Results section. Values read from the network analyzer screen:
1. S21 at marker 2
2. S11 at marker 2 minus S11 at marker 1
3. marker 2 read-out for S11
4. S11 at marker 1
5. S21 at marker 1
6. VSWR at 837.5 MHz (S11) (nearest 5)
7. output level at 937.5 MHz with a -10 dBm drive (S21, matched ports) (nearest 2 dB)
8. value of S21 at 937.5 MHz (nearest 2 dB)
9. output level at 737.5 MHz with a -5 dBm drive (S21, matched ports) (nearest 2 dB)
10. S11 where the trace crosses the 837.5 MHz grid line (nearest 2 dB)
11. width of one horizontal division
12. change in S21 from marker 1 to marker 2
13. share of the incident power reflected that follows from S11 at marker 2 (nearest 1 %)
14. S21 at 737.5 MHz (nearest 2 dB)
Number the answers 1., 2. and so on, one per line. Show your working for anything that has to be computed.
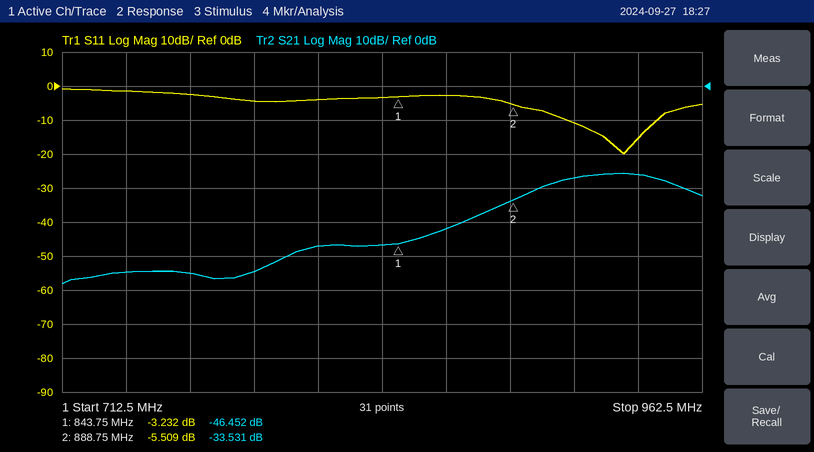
1. -33.531 dB
2. -5.509 − (-3.232) = -2.277 dB
3. -5.509 dB
4. -3.232 dB
5. -46.452 dB
6. |Γ| = 10^(-4/20) = 0.6310; VSWR = (1 + 0.6310)/(1 − 0.6310) ≈ 4.42, so 5 to the nearest 5
7. -10 dBm + (-26 dB) = -36 dBm
8. -26 dB
9. -5 dBm + (-54 dB) = -60 dBm
10. -4 dB
11. 25 MHz
12. -33.531 − (-46.452) = 12.921 dB
13. 10^(-5.509/10) ≈ 28 %
14. -54 dB
